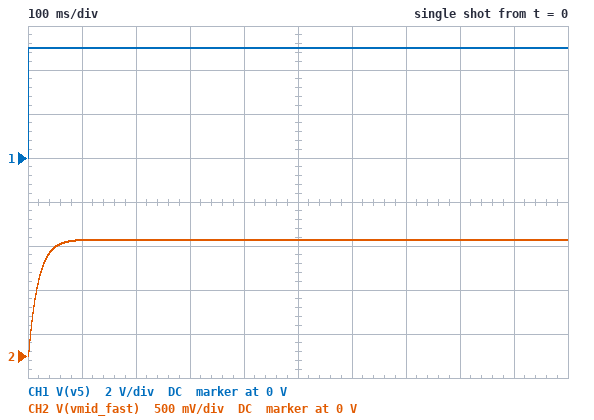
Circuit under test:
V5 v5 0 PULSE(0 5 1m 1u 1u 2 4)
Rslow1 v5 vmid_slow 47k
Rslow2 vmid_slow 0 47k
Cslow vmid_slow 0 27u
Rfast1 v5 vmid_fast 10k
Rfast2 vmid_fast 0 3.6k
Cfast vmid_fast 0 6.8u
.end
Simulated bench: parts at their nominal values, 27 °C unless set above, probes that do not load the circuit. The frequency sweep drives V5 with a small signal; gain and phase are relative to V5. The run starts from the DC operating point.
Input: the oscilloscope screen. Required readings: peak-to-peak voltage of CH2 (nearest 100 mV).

1.3 V
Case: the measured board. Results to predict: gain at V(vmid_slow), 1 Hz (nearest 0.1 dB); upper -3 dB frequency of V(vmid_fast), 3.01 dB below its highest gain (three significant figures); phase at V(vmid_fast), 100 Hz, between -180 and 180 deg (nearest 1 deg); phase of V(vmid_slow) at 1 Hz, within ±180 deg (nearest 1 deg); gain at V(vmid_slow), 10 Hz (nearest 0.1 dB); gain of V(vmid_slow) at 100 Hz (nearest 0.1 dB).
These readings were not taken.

-18.3 dB
8.84 Hz
-85 deg
-76 deg
-38.0 dB
-58.0 dB
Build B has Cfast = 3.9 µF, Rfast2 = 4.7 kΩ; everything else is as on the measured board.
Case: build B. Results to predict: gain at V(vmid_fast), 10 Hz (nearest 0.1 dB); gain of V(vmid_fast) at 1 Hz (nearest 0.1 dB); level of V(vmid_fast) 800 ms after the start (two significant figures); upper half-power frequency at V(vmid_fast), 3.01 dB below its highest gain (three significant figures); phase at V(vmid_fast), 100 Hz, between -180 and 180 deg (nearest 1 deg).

-12.0 dB
-9.9 dB
1.6 V
12.8 Hz
-83 deg
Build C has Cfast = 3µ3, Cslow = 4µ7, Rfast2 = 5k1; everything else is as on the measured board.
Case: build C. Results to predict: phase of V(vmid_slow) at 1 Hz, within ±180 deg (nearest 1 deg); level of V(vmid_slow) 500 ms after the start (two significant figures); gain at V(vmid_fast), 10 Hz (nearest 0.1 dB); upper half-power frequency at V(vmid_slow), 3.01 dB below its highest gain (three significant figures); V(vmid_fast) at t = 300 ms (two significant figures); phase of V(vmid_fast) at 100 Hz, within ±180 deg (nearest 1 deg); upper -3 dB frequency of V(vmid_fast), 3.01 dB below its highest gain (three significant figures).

-35 deg
2.5 V
-11.2 dB
1.44 Hz
1.7 V
-82 deg
14.3 Hz
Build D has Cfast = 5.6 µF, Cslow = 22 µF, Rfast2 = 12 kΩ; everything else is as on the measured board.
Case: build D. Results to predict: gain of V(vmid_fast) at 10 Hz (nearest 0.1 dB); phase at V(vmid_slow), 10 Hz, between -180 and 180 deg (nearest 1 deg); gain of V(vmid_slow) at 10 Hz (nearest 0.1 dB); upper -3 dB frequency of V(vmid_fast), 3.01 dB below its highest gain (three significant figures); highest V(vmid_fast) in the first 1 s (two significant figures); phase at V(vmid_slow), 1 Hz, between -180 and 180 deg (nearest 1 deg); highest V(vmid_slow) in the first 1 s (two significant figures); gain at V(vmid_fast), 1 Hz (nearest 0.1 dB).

-12.0 dB
-88 deg
-36.3 dB
5.21 Hz
2.7 V
-73 deg
2.1 V
-5.4 dB
